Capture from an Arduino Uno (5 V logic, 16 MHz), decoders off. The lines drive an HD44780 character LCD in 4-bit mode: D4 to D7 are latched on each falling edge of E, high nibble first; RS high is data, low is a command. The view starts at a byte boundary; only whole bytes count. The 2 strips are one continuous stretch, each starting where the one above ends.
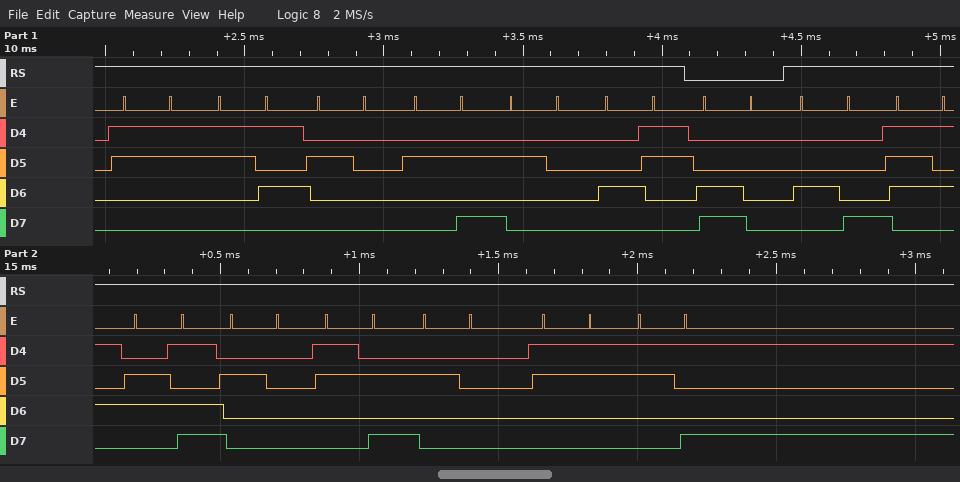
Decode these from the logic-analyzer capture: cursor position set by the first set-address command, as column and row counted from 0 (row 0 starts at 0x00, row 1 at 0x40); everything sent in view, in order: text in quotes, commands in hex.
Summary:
column 0, row 1
"35 * C" 0xC0 "Hum : 39"
